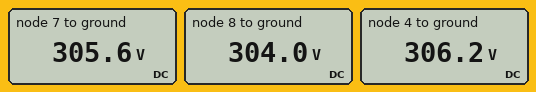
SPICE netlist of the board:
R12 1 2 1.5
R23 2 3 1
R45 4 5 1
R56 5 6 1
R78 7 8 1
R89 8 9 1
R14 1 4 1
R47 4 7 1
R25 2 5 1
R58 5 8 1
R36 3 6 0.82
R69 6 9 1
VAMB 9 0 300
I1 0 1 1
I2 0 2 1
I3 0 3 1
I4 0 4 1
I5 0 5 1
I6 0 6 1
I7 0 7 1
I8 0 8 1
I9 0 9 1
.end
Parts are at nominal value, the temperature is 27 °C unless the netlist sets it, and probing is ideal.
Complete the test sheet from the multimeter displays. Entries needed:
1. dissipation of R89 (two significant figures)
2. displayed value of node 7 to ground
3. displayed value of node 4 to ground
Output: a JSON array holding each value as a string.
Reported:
["16 W", "305.6 V", "306.2 V"]
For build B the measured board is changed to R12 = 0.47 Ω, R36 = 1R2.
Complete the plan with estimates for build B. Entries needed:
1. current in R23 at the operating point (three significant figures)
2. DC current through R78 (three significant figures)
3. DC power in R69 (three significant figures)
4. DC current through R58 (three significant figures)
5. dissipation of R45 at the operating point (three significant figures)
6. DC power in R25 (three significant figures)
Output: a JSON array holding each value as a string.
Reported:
["559 mA", "1.61 A", "15.9 W", "1.40 A", "682 mW", "1.00 W"]
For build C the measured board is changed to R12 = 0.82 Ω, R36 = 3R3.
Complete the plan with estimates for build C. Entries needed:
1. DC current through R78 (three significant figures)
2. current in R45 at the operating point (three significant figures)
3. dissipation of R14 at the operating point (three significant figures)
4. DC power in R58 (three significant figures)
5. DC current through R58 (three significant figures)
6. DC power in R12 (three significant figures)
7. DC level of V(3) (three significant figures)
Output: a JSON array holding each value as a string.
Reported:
["1.71 A", "956 mA", "448 mW", "2.16 W", "1.47 A", "89.5 mW", "307 V"]
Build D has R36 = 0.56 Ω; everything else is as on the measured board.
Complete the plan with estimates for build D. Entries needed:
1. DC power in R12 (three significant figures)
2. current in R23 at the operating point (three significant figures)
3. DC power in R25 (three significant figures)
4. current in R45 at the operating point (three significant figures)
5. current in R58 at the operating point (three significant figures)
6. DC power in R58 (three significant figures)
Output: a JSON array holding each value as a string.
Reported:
["368 mW", "841 mA", "429 mW", "893 mA", "1.33 A", "1.77 W"]
